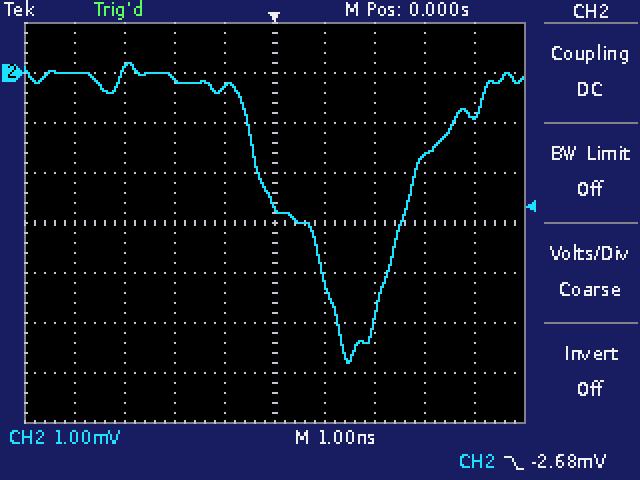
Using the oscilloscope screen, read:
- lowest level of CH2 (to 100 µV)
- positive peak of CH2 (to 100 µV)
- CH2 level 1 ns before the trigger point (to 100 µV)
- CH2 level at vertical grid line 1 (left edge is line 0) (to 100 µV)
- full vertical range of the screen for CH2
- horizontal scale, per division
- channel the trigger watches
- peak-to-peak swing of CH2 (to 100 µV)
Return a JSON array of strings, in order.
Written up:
["-5.8 mV", "200 µV", "-300 µV", "0.0 mV", "8 mV", "1 ns", "CH2", "6.0 mV"]
